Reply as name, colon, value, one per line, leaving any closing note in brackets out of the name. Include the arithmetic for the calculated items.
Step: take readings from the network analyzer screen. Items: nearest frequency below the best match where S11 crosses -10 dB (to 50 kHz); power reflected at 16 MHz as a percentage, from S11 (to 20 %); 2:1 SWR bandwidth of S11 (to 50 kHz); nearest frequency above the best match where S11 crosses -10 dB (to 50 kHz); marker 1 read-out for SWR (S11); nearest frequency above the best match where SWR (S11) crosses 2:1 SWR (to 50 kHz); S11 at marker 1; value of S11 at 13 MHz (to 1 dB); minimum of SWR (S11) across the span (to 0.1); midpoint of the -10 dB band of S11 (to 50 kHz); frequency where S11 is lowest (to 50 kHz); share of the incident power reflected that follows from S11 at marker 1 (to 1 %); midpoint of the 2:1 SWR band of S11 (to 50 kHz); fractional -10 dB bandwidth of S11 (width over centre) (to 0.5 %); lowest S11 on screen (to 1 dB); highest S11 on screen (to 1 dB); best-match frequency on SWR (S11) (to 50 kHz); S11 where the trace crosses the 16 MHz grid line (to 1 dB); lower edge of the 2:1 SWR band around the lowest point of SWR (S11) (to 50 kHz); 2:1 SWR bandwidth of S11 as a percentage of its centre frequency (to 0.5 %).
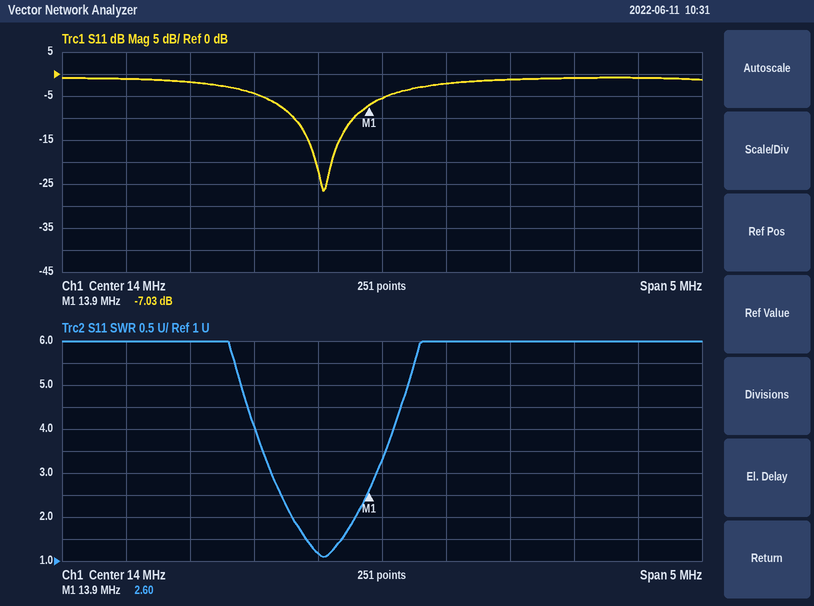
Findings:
nearest frequency below the best match where S11 crosses -10 dB: 13.30 MHz
power reflected at 16 MHz as a percentage, from S11: 10^(-1/10) ≈ 79.4 %, so 80 % to the nearest 20 %
2:1 SWR bandwidth of S11: 13.80 MHz − 13.30 MHz = 500 kHz
nearest frequency above the best match where S11 crosses -10 dB: 13.80 MHz
marker 1 read-out for SWR: 2.60
nearest frequency above the best match where SWR (S11) crosses 2:1 SWR: 13.80 MHz
S11 at marker 1: -7.03 dB
value of S11 at 13 MHz: -4 dB
minimum of SWR (S11) across the span: 1.1
midpoint of the -10 dB band of S11: 13.55 MHz
frequency where S11 is lowest: 13.55 MHz
share of the incident power reflected that follows from S11 at marker 1: 10^(-7.03/10) ≈ 20 %
midpoint of the 2:1 SWR band of S11: 13.55 MHz
fractional -10 dB bandwidth of S11 (width over centre): 500 kHz / 13.55 MHz ≈ 3.69 %, so 3.5 % to the nearest 0.5 %
lowest S11 on screen: -27 dB
highest S11 on screen: -1 dB
best-match frequency on SWR (S11): 13.55 MHz
S11 where the trace crosses the 16 MHz grid line: -1 dB
lower edge of the 2:1 SWR band around the lowest point of SWR (S11): 13.30 MHz
2:1 SWR bandwidth of S11 as a percentage of its centre frequency: 500 kHz / 13.55 MHz ≈ 3.69 %, so 3.5 % to the nearest 0.5 %
